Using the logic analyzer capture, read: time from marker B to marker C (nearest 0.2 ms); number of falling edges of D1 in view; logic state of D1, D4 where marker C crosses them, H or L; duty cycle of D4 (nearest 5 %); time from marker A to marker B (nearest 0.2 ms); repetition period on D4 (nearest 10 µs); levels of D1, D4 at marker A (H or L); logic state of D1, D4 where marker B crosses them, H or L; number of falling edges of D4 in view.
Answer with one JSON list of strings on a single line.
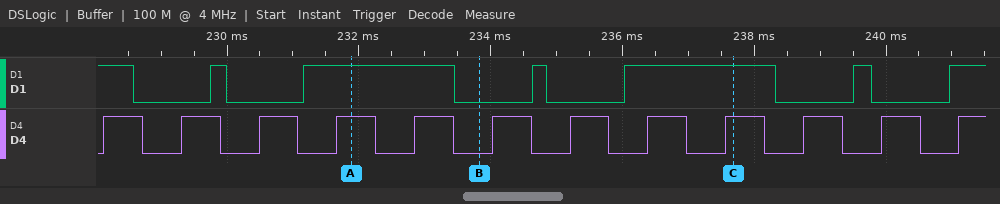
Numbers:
["3.8 ms", "6", "D1=H, D4=H", "50 %", "2 ms", "1180 µs", "D1=H, D4=H", "D1=L, D4=L", "11"]
